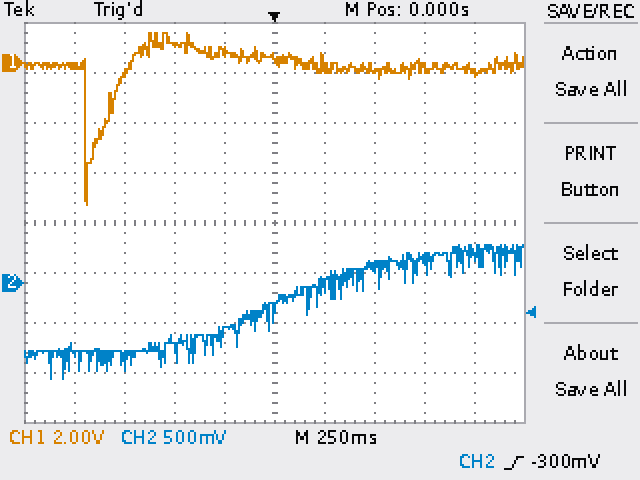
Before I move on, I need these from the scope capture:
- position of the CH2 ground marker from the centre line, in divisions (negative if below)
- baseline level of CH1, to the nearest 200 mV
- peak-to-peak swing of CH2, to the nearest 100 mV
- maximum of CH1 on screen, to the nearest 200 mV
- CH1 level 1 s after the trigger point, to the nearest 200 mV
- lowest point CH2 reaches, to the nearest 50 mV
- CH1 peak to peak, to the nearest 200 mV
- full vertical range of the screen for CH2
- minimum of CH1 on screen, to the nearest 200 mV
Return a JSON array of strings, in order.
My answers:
["-1.2 div", "-200 mV", "1.30 V", "1.2 V", "-400 mV", "-950 mV", "6.8 V", "4 V", "-5.6 V"]
